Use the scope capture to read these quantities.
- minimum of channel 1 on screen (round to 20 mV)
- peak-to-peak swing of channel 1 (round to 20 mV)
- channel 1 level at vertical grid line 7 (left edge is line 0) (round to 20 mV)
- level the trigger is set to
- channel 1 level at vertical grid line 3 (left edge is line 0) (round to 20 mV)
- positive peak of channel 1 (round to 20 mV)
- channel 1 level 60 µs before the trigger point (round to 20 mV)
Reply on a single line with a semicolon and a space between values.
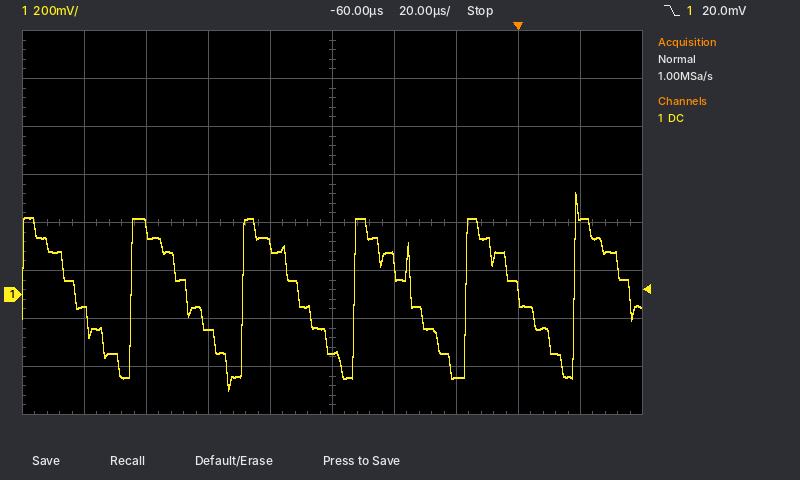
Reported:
-400 mV; 820 mV; -340 mV; 20.0 mV; -140 mV; 420 mV; -240 mV
